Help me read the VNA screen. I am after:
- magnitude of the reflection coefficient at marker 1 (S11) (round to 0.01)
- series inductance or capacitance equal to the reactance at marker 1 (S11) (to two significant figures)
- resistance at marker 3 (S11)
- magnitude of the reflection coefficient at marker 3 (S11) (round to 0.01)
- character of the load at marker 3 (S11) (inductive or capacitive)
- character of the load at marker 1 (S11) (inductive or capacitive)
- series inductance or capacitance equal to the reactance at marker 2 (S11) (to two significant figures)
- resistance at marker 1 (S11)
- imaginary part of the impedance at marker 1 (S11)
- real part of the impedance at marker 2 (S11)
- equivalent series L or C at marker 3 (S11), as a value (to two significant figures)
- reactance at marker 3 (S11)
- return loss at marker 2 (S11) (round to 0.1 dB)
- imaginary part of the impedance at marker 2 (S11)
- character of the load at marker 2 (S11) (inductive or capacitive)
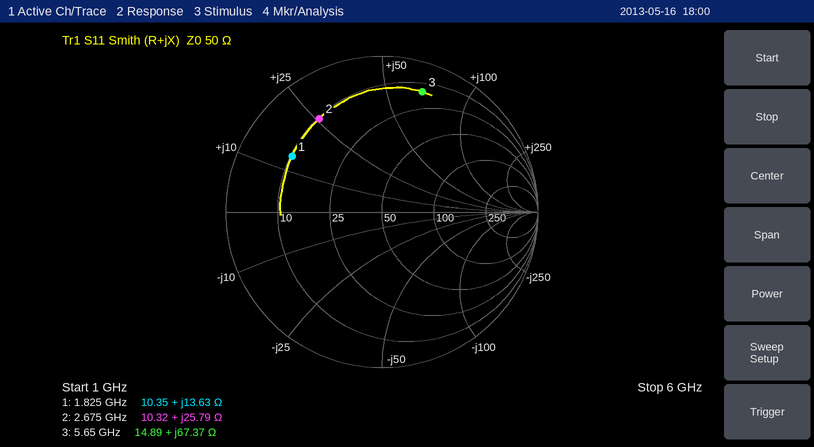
0.68
1.2 nH
14.89 Ω
0.81
inductive
inductive
1.5 nH
10.35 Ω
+13.63 Ω
10.32 Ω
1.9 nH
+67.37 Ω
2.8 dB
+25.79 Ω
inductive
